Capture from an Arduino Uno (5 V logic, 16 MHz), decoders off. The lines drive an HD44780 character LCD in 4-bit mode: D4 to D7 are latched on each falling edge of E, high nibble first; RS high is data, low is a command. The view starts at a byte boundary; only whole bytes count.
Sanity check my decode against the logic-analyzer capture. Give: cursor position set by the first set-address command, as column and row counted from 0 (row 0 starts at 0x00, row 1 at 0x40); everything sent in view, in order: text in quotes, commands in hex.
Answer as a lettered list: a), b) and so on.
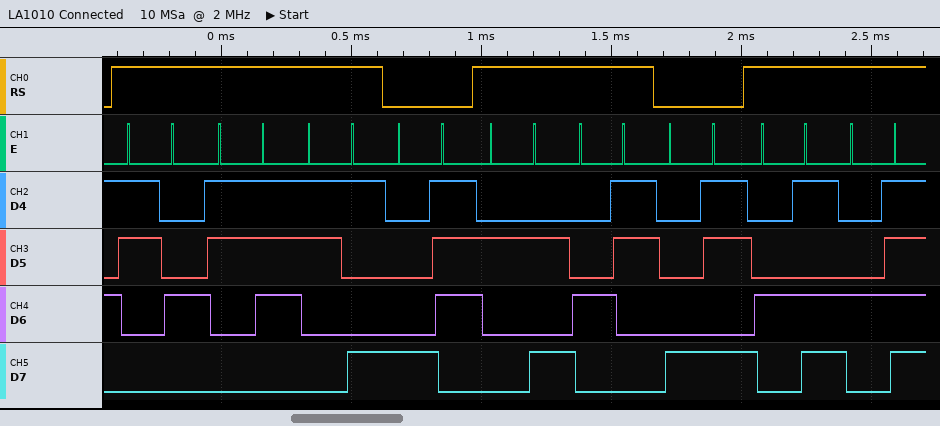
a) column 7, row 0
b) "479" 0x87 "*C" 0x8B "MO"
